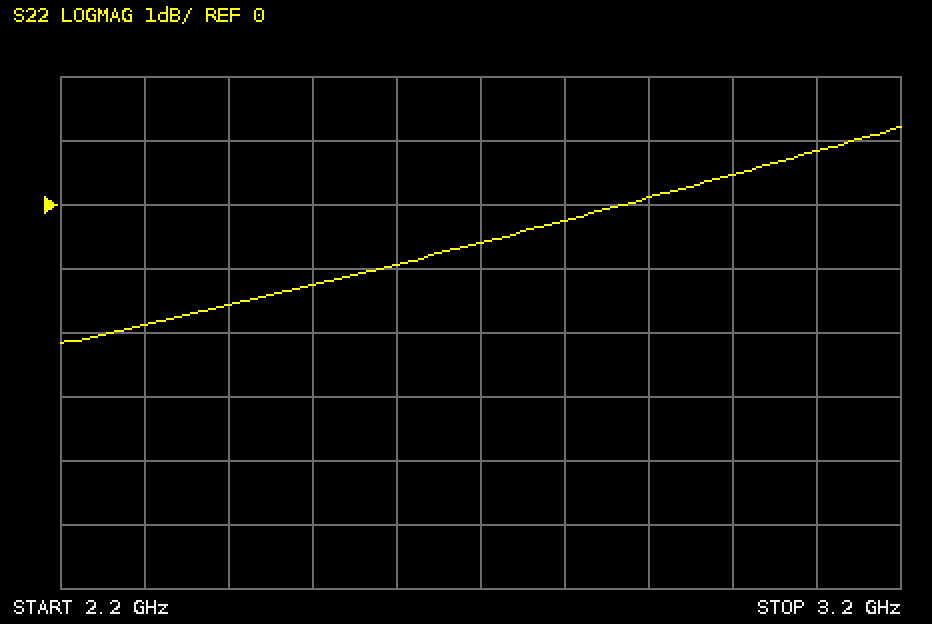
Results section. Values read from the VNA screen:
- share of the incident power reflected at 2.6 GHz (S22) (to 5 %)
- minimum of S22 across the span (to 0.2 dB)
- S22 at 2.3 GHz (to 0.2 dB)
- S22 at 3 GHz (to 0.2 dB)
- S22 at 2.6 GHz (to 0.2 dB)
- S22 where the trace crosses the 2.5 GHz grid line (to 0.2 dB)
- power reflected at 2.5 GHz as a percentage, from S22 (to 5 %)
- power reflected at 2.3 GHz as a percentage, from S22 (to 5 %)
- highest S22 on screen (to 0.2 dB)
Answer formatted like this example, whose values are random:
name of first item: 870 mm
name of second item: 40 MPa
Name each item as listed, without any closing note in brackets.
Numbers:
share of the incident power reflected at 2.6 GHz (S22): 80 %
minimum of S22 across the span: -2.2 dB
S22 at 2.3 GHz: -1.8 dB
S22 at 3 GHz: 0.4 dB
S22 at 2.6 GHz: -1.0 dB
S22 where the trace crosses the 2.5 GHz grid line: -1.2 dB
power reflected at 2.5 GHz as a percentage, from S22: 75 %
power reflected at 2.3 GHz as a percentage, from S22: 65 %
highest S22 on screen: 1.2 dB
